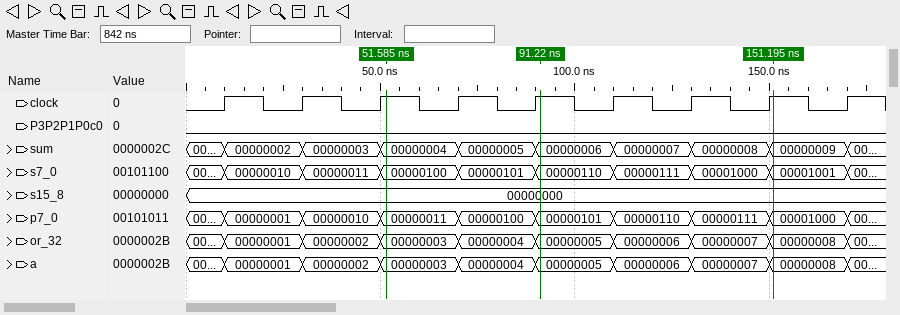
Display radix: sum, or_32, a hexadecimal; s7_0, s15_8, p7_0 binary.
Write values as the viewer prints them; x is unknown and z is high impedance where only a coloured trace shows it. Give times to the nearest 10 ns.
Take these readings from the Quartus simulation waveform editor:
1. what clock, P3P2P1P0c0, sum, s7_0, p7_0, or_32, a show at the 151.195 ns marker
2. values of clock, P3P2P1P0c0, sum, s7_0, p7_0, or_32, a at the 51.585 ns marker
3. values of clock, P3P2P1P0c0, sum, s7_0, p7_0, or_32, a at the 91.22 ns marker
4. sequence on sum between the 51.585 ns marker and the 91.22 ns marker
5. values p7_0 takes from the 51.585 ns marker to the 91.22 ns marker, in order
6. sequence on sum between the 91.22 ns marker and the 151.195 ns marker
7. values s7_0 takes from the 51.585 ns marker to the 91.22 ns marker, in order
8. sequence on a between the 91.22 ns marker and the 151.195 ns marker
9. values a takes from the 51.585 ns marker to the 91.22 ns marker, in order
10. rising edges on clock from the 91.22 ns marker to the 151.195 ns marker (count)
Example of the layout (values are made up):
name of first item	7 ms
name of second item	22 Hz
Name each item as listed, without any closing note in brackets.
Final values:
what clock, P3P2P1P0c0, sum, s7_0, p7_0, or_32, a show at the 151.195 ns marker	clock=1, P3P2P1P0c0=0, sum=00000009, s7_0=00001001, p7_0=00001000, or_32=00000008, a=00000008
values of clock, P3P2P1P0c0, sum, s7_0, p7_0, or_32, a at the 51.585 ns marker	clock=1, P3P2P1P0c0=0, sum=00000004, s7_0=00000100, p7_0=00000011, or_32=00000003, a=00000003
values of clock, P3P2P1P0c0, sum, s7_0, p7_0, or_32, a at the 91.22 ns marker	clock=1, P3P2P1P0c0=0, sum=00000006, s7_0=00000110, p7_0=00000101, or_32=00000005, a=00000005
sequence on sum between the 51.585 ns marker and the 91.22 ns marker	00000004, 00000005, 00000006
values p7_0 takes from the 51.585 ns marker to the 91.22 ns marker, in order	00000011, 00000100, 00000101
sequence on sum between the 91.22 ns marker and the 151.195 ns marker	00000006, 00000007, 00000008, 00000009
values s7_0 takes from the 51.585 ns marker to the 91.22 ns marker, in order	00000100, 00000101, 00000110
sequence on a between the 91.22 ns marker and the 151.195 ns marker	00000005, 00000006, 00000007, 00000008
values a takes from the 51.585 ns marker to the 91.22 ns marker, in order	00000003, 00000004, 00000005
rising edges on clock from the 91.22 ns marker to the 151.195 ns marker	3
